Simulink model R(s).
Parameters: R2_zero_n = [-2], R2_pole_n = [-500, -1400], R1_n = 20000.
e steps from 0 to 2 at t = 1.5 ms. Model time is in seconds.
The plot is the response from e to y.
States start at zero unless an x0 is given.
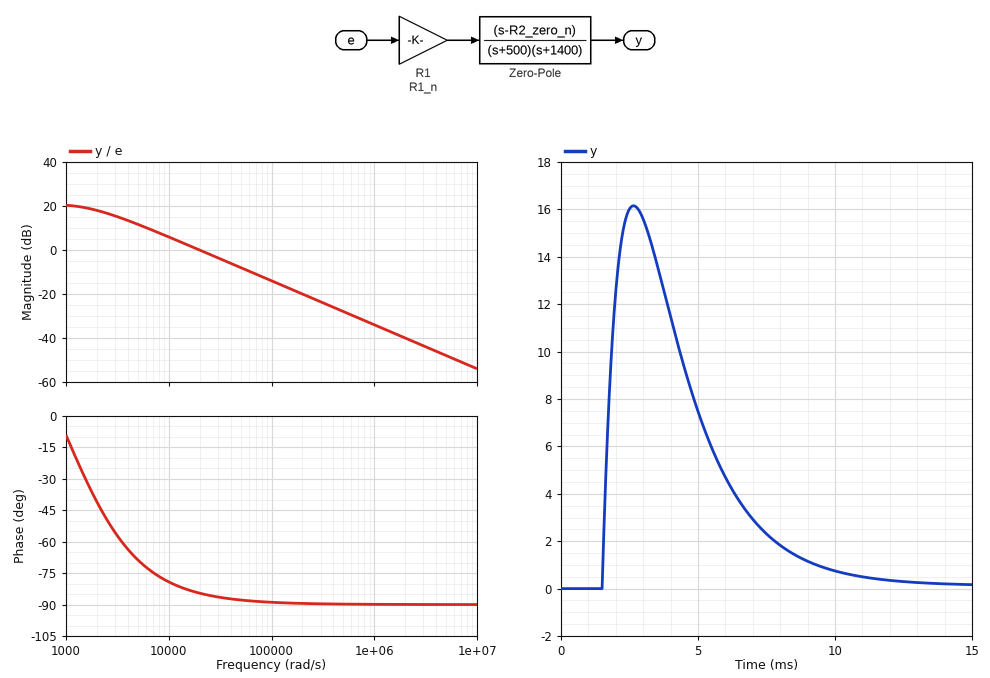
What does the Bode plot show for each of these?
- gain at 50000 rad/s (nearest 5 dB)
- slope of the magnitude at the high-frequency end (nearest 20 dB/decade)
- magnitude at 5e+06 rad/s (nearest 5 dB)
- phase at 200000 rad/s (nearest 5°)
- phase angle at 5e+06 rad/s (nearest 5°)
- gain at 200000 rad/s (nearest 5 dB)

-10 dB
-20 dB/decade
-50 dB
-90°
-90°
-20 dB
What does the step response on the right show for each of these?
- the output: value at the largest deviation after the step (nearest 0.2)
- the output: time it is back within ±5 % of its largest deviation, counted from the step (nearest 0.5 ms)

16.2
8.0 ms
